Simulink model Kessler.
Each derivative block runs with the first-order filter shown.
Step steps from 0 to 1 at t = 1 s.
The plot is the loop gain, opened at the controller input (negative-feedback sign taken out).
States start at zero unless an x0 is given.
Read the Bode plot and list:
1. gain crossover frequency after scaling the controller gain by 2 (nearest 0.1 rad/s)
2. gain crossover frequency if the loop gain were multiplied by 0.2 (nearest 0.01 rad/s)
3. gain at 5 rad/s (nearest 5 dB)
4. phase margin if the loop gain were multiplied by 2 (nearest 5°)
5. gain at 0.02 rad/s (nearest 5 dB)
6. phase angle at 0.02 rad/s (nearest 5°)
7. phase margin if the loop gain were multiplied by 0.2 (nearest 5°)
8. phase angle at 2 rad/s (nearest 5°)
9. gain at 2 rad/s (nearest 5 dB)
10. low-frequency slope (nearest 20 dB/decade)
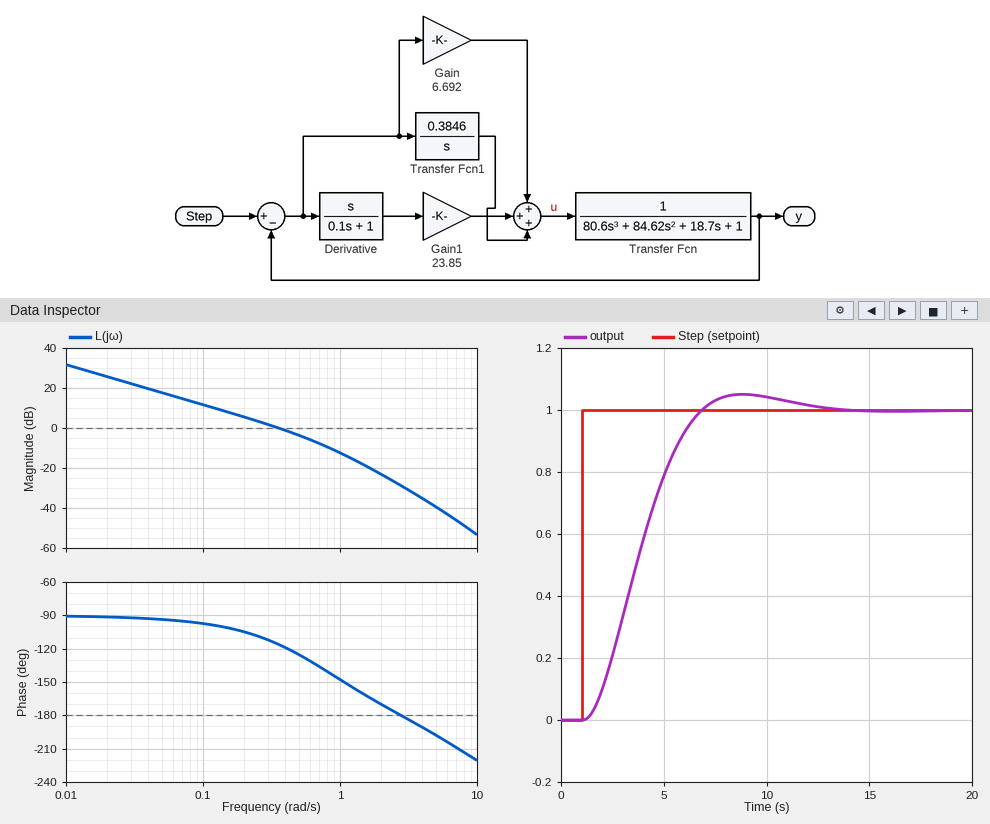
0.6 rad/s
0.08 rad/s
-40 dB
50°
25 dB
-90°
85°
-170°
-25 dB
-20 dB/decade
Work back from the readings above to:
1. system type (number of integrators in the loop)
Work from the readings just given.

1
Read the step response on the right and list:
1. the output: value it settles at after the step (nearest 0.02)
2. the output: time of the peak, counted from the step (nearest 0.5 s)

1.00
8.0 s
